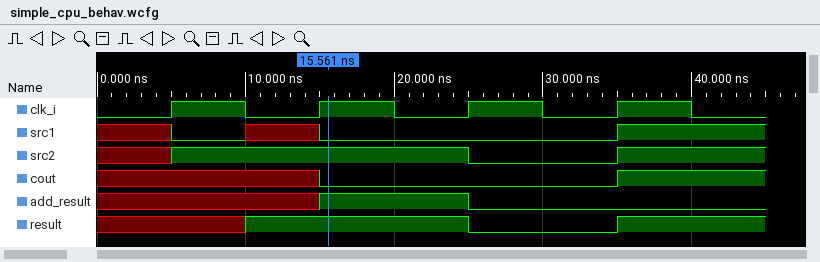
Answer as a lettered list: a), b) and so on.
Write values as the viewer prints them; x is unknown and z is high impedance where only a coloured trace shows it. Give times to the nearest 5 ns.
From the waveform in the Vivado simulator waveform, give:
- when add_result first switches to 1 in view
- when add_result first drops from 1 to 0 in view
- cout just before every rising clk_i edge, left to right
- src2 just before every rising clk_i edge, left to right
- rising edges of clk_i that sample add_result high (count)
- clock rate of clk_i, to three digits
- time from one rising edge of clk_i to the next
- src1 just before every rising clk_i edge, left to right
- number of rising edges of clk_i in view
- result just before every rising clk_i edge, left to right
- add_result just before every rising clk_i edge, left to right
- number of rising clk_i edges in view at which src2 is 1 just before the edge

a) 15 ns
b) 25 ns
c) x x 0 0
d) x 1 1 0
e) 1
f) 100 MHz
g) 10 ns
h) x x 0 0
i) 4
j) x 1 1 0
k) x x 1 0
l) 2
